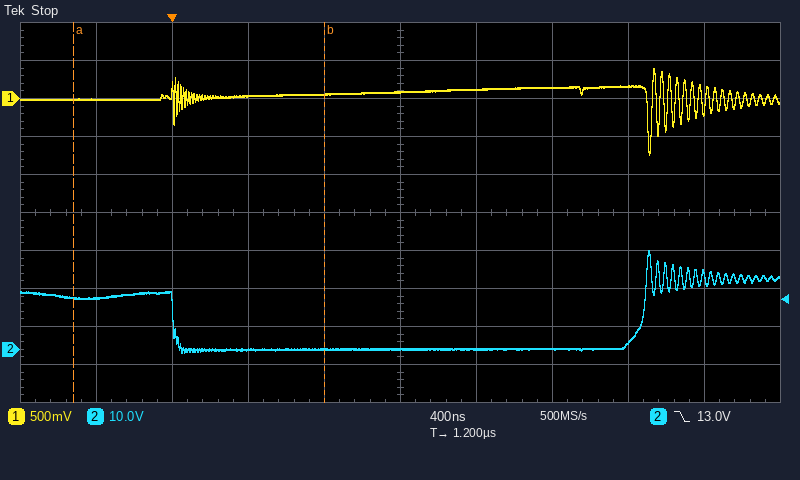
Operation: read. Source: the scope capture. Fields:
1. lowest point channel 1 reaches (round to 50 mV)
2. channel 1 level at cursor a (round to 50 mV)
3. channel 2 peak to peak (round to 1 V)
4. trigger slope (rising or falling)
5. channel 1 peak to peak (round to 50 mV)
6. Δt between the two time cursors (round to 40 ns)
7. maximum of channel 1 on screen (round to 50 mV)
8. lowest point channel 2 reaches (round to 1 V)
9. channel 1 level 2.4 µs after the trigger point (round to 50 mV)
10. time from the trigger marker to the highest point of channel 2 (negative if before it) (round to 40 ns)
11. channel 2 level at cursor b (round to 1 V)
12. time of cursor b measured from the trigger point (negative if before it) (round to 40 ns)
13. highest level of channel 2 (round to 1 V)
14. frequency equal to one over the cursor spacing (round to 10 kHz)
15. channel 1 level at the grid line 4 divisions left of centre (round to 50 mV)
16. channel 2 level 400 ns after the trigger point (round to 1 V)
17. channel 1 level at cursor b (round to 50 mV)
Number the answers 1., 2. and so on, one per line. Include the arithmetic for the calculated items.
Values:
1. -750 mV
2. 0 mV
3. 26 V − (-1 V) = 27 V
4. falling
5. 400 mV − (-750 mV) = 1.15 V
6. 1.32 µs
7. 400 mV
8. -1 V
9. 150 mV
10. +2.52 µs
11. 0 V
12. +800 ns
13. 26 V
14. 1 / 1.32 µs ≈ 760 kHz
15. 0 mV
16. 0 V
17. 50 mV
